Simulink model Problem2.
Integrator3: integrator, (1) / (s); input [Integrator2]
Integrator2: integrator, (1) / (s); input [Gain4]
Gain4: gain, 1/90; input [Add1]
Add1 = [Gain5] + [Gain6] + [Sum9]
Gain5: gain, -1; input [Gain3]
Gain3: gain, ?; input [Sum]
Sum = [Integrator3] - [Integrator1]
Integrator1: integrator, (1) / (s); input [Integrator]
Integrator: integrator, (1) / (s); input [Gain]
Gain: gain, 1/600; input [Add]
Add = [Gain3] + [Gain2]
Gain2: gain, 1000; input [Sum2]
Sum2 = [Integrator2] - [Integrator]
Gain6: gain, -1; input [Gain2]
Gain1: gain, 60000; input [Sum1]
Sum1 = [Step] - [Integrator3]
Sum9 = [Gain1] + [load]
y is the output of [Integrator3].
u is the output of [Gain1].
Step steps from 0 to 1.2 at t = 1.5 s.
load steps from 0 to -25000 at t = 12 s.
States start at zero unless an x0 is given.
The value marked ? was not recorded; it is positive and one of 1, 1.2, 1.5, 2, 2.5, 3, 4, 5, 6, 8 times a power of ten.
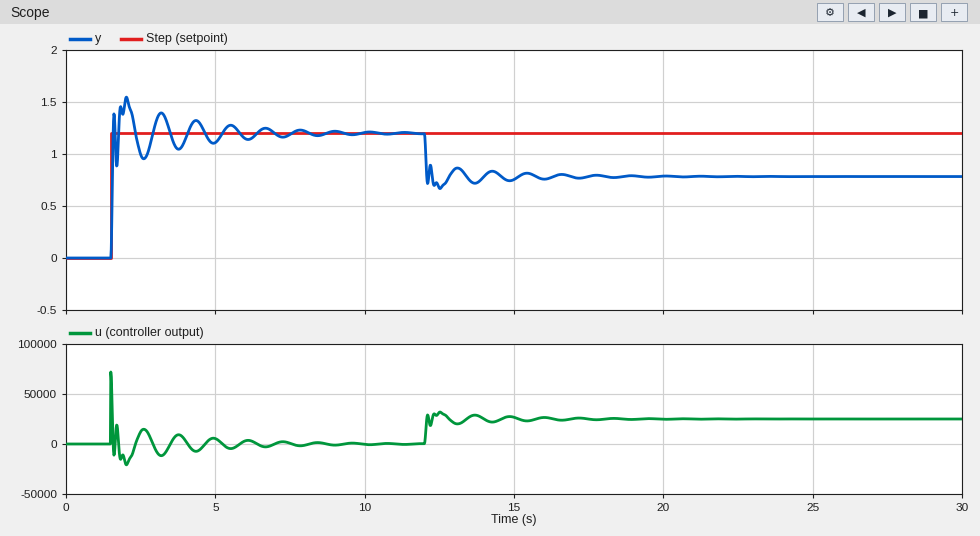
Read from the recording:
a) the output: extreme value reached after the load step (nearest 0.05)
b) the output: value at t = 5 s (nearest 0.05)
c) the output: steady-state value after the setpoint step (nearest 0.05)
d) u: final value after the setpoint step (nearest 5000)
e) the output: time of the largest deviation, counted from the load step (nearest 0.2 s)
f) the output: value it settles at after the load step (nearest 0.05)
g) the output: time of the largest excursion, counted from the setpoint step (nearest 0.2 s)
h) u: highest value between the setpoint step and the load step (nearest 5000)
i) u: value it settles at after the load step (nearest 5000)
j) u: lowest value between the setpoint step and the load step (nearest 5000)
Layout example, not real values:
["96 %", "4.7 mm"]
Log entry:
["0.65", "1.10", "1.20", "0", "0.6 s", "0.80", "0.6 s", "70000", "25000", "-20000"]
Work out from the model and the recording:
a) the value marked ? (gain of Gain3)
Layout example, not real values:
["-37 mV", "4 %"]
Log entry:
["25000"]
